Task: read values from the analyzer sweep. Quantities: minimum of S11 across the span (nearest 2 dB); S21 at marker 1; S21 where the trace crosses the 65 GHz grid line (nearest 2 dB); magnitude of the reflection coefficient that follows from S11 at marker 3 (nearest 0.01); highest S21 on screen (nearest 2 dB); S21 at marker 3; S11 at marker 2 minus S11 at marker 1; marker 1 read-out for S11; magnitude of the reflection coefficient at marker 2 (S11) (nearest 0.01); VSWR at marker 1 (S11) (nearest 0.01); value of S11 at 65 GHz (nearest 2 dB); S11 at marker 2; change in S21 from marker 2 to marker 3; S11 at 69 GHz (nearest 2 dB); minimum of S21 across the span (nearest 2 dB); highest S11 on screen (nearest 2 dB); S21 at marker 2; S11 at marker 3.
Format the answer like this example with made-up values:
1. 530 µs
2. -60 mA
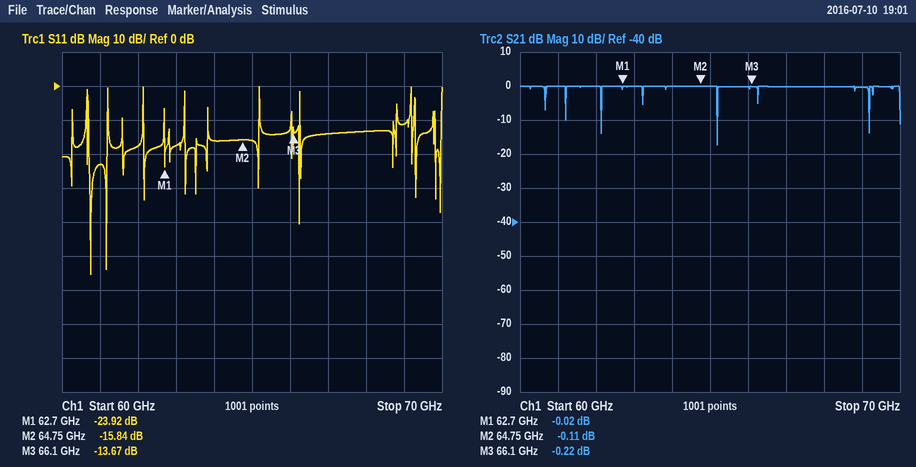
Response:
1. -56 dB
2. -0.02 dB
3. 0 dB
4. 0.21
5. 0 dB
6. -0.22 dB
7. 8.08 dB
8. -23.92 dB
9. 0.16
10. 1.14
11. -16 dB
12. -15.84 dB
13. -0.11 dB
14. -12 dB
15. -18 dB
16. 0 dB
17. -0.11 dB
18. -13.67 dB
